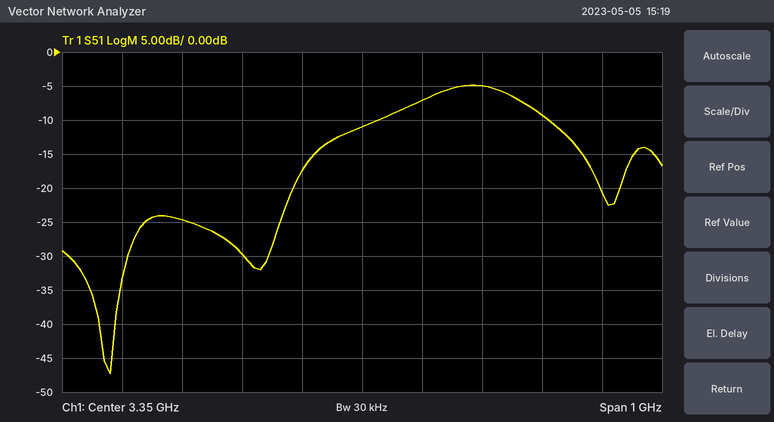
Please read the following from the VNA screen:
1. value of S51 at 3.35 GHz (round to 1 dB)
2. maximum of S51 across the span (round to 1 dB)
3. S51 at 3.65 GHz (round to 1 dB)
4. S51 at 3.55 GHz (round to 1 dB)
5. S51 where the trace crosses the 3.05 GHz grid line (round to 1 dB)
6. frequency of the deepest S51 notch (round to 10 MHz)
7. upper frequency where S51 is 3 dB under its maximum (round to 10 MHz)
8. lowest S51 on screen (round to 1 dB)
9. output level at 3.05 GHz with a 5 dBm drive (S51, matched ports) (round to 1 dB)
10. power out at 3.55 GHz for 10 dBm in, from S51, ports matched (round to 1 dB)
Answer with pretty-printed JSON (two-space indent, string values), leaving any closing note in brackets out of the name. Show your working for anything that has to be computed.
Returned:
{
  "value of S51 at 3.35 GHz": "-11 dB",
  "maximum of S51 across the span": "-5 dB",
  "S51 at 3.65 GHz": "-9 dB",
  "S51 at 3.55 GHz": "-5 dB",
  "S51 where the trace crosses the 3.05 GHz grid line": "-25 dB",
  "frequency of the deepest S51 notch": "2.93 GHz",
  "upper frequency where S51 is 3 dB under its maximum": "3.63 GHz",
  "lowest S51 on screen": "-47 dB",
  "output level at 3.05 GHz with a 5 dBm drive (S51, matched ports)": "5 dBm + (-25 dB) = -20 dBm",
  "power out at 3.55 GHz for 10 dBm in, from S51, ports matched": "10 dBm + (-5 dB) = 5 dBm"
}
